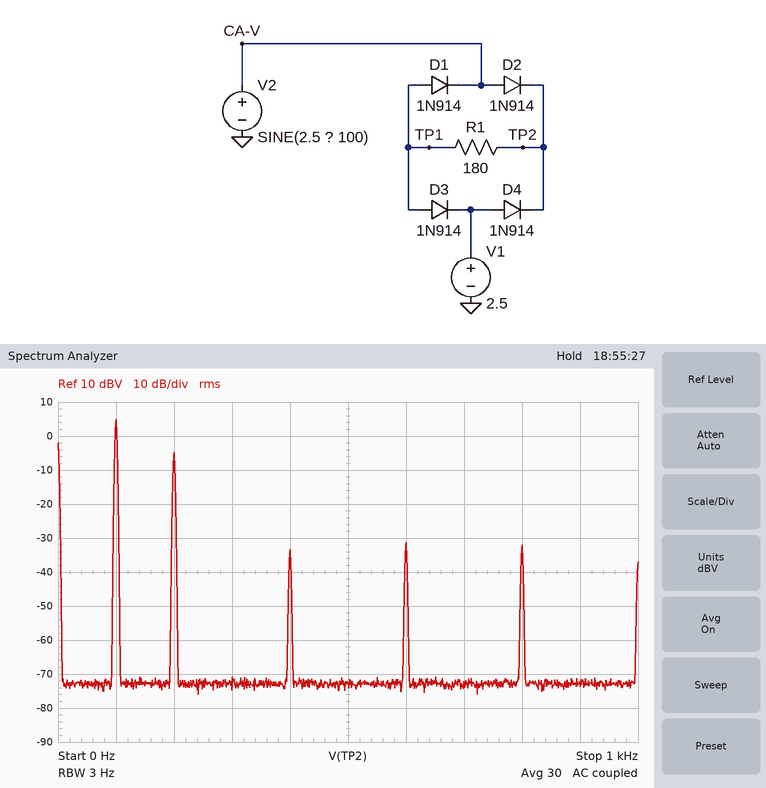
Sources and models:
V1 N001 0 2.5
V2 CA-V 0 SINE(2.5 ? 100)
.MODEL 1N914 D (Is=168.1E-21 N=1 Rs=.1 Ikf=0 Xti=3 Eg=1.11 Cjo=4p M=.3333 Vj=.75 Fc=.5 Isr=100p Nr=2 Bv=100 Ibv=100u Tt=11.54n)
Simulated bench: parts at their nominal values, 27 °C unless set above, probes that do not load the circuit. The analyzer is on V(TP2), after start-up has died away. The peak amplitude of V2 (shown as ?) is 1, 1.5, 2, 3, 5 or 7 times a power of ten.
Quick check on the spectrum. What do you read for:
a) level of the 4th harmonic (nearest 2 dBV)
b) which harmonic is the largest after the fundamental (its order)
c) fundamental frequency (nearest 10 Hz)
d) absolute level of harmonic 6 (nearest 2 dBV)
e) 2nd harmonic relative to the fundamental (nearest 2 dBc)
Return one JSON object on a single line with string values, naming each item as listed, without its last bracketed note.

{"level of the 4th harmonic": "-34 dBV", "which harmonic is the largest after the fundamental": "2", "fundamental frequency": "100 Hz", "absolute level of harmonic 6": "-32 dBV", "2nd harmonic relative to the fundamental": "-10 dBc"}
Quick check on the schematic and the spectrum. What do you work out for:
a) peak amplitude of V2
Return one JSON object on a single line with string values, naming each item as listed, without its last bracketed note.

{"peak amplitude of V2": "5 V"}
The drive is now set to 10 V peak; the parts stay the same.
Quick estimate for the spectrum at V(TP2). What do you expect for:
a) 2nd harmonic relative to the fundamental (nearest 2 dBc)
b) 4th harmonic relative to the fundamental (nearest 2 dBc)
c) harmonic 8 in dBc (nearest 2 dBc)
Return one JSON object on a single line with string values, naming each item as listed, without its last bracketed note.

{"2nd harmonic relative to the fundamental": "-8 dBc", "4th harmonic relative to the fundamental": "-24 dBc", "harmonic 8 in dBc": "-54 dBc"}
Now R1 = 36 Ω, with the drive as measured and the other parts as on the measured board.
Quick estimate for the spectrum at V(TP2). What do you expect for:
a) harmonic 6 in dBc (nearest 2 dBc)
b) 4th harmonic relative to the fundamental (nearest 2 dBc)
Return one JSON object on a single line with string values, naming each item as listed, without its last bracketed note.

{"harmonic 6 in dBc": "-34 dBc", "4th harmonic relative to the fundamental": "-46 dBc"}
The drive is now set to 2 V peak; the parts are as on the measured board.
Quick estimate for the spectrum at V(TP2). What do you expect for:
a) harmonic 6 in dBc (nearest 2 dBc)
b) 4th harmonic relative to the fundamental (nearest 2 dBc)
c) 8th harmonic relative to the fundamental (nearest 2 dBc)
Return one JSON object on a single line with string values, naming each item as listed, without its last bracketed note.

{"harmonic 6 in dBc": "-42 dBc", "4th harmonic relative to the fundamental": "-30 dBc", "8th harmonic relative to the fundamental": "-56 dBc"}
